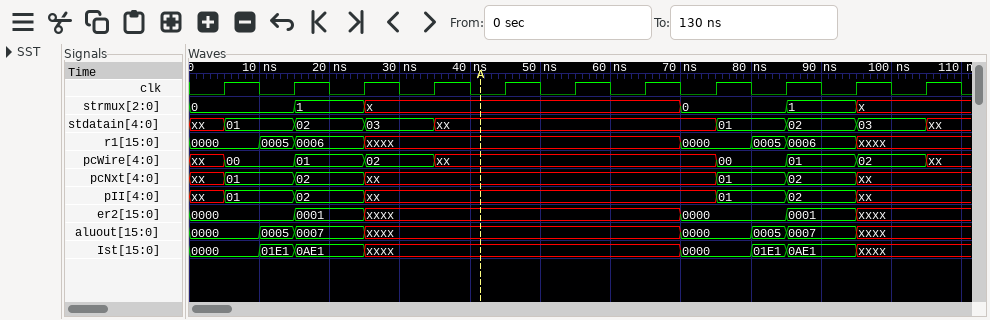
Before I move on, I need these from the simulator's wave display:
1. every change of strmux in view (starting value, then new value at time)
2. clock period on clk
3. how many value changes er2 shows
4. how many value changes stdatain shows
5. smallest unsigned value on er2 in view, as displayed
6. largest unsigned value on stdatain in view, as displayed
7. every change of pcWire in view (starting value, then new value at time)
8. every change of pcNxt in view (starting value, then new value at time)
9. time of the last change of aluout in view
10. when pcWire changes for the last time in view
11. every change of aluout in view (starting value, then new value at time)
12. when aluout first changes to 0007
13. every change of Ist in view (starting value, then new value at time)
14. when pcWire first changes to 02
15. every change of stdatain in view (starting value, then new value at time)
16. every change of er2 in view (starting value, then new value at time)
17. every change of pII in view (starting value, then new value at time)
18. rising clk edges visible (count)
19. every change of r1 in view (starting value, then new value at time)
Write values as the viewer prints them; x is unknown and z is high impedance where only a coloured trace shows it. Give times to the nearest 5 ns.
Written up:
0, 1 at 15 ns, x at 25 ns, 0 at 70 ns, 1 at 85 ns, x at 95 ns
10 ns
5
8
0000
03
xx, 00 at 5 ns, 01 at 15 ns, 02 at 25 ns, xx at 35 ns, 00 at 75 ns, 01 at 85 ns, 02 at 95 ns, xx at 105 ns
xx, 01 at 5 ns, 02 at 15 ns, xx at 25 ns, 01 at 75 ns, 02 at 85 ns, xx at 95 ns
95 ns
105 ns
0000, 0005 at 10 ns, 0007 at 15 ns, xxxx at 25 ns, 0000 at 70 ns, 0005 at 80 ns, 0007 at 85 ns, xxxx at 95 ns
15 ns
0000, 01E1 at 10 ns, 0AE1 at 15 ns, xxxx at 25 ns, 0000 at 70 ns, 01E1 at 80 ns, 0AE1 at 85 ns, xxxx at 95 ns
25 ns
xx, 01 at 5 ns, 02 at 15 ns, 03 at 25 ns, xx at 35 ns, 01 at 75 ns, 02 at 85 ns, 03 at 95 ns, xx at 105 ns
0000, 0001 at 15 ns, xxxx at 25 ns, 0000 at 70 ns, 0001 at 85 ns, xxxx at 95 ns
xx, 01 at 5 ns, 02 at 15 ns, xx at 25 ns, 01 at 75 ns, 02 at 85 ns, xx at 95 ns
11
0000, 0005 at 10 ns, 0006 at 15 ns, xxxx at 25 ns, 0000 at 70 ns, 0005 at 80 ns, 0006 at 85 ns, xxxx at 95 ns
